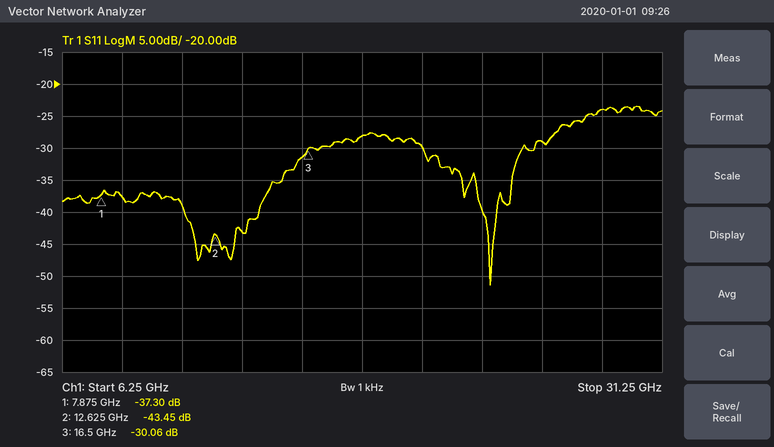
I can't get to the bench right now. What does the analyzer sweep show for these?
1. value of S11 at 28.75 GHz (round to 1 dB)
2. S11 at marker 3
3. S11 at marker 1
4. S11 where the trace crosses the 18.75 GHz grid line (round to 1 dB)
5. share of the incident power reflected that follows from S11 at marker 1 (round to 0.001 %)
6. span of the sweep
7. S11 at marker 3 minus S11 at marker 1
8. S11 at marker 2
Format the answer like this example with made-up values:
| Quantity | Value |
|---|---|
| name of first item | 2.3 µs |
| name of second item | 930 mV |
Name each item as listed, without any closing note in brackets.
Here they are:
| Quantity | Value |
|---|---|
| value of S11 at 28.75 GHz | -24 dB |
| S11 at marker 3 | -30.06 dB |
| S11 at marker 1 | -37.30 dB |
| S11 where the trace crosses the 18.75 GHz grid line | -28 dB |
| share of the incident power reflected that follows from S11 at marker 1 | 0.019 % |
| span of the sweep | 25 GHz |
| S11 at marker 3 minus S11 at marker 1 | 7.24 dB |
| S11 at marker 2 | -43.45 dB |
